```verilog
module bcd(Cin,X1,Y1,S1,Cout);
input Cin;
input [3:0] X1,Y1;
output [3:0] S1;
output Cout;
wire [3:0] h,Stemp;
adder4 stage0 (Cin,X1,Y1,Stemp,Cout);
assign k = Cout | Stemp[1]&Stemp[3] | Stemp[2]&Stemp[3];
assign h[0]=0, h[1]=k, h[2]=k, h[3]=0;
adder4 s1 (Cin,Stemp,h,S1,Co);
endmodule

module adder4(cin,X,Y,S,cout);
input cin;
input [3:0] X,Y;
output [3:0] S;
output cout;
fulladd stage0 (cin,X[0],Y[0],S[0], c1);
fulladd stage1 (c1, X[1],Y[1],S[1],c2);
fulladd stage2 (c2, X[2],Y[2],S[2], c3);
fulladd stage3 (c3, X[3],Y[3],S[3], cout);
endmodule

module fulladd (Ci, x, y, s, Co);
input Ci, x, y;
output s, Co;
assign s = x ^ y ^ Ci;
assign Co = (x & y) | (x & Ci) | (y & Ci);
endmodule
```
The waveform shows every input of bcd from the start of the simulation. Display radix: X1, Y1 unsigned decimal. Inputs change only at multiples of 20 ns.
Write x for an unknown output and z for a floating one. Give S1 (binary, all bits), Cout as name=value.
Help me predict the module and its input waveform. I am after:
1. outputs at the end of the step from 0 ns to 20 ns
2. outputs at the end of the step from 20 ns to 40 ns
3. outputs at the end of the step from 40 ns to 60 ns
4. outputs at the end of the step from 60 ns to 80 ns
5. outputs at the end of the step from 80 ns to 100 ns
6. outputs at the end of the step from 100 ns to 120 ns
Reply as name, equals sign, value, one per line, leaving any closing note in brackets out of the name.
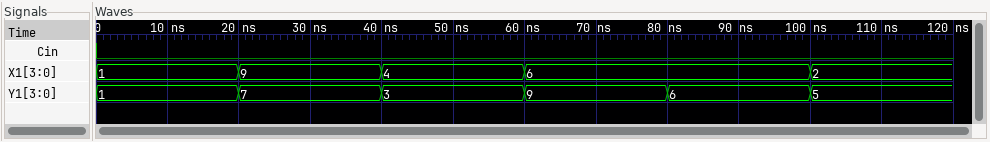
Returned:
outputs at the end of the step from 0 ns to 20 ns = S1=0010, Cout=0
outputs at the end of the step from 20 ns to 40 ns = S1=0110, Cout=1
outputs at the end of the step from 40 ns to 60 ns = S1=0111, Cout=0
outputs at the end of the step from 60 ns to 80 ns = S1=0101, Cout=0
outputs at the end of the step from 80 ns to 100 ns = S1=0010, Cout=0
outputs at the end of the step from 100 ns to 120 ns = S1=0111, Cout=0
